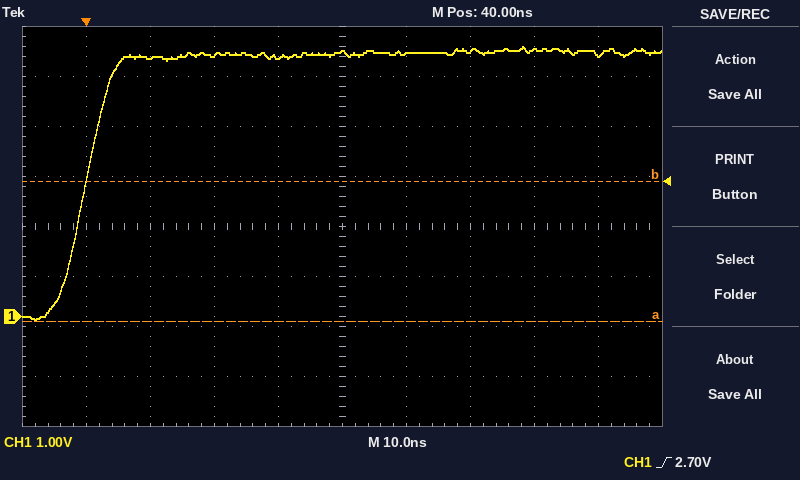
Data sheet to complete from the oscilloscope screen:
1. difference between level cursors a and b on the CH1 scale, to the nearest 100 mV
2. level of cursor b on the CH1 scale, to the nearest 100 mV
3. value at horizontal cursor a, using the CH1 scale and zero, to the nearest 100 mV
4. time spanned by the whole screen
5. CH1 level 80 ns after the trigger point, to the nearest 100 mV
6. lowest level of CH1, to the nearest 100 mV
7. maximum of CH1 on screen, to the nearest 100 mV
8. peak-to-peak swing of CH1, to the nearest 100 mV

2.8 V
2.7 V
-100 mV
100 ns
5.2 V
-100 mV
5.4 V
5.5 V
